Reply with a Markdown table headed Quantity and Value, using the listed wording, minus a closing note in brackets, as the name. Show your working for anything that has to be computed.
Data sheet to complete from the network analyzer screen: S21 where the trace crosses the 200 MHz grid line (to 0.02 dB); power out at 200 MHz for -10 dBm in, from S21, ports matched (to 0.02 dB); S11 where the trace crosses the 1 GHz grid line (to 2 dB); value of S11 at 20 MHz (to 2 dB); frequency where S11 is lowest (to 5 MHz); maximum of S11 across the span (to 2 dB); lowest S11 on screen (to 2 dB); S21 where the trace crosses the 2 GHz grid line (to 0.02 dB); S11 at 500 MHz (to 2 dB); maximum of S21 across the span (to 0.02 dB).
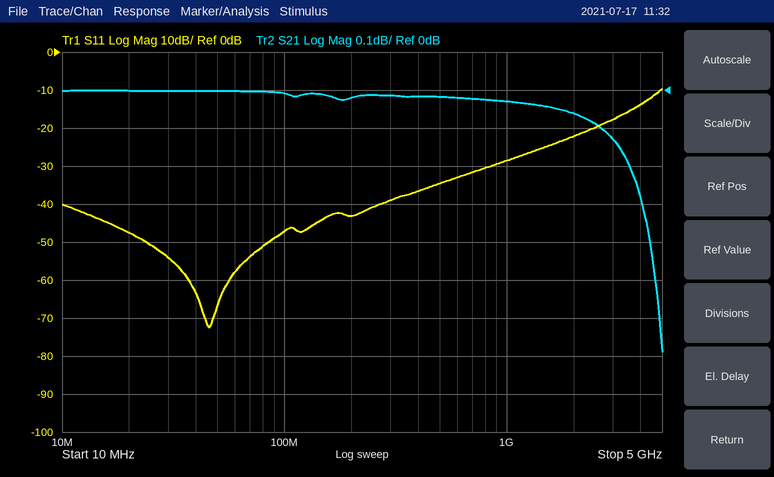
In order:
| Quantity | Value |
|---|---|
| S21 where the trace crosses the 200 MHz grid line | -0.02 dB |
| power out at 200 MHz for -10 dBm in, from S21, ports matched | -10 dBm + (-0.02 dB) = -10.02 dBm |
| S11 where the trace crosses the 1 GHz grid line | -28 dB |
| value of S11 at 20 MHz | -48 dB |
| frequency where S11 is lowest | 45 MHz |
| maximum of S11 across the span | -10 dB |
| lowest S11 on screen | -72 dB |
| S21 where the trace crosses the 2 GHz grid line | -0.06 dB |
| S11 at 500 MHz | -34 dB |
| maximum of S21 across the span | 0.00 dB |
